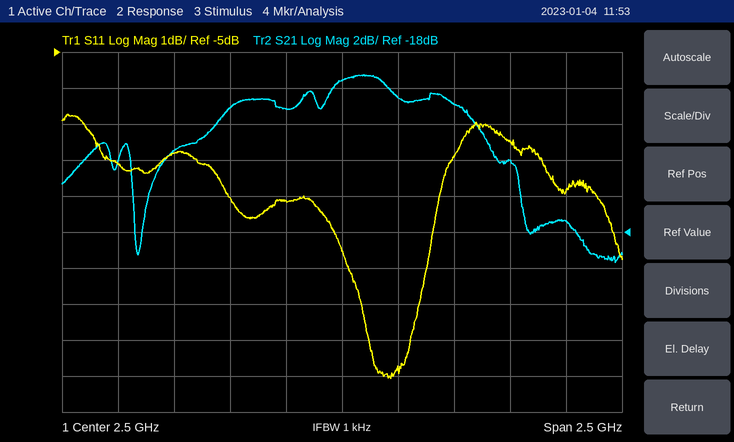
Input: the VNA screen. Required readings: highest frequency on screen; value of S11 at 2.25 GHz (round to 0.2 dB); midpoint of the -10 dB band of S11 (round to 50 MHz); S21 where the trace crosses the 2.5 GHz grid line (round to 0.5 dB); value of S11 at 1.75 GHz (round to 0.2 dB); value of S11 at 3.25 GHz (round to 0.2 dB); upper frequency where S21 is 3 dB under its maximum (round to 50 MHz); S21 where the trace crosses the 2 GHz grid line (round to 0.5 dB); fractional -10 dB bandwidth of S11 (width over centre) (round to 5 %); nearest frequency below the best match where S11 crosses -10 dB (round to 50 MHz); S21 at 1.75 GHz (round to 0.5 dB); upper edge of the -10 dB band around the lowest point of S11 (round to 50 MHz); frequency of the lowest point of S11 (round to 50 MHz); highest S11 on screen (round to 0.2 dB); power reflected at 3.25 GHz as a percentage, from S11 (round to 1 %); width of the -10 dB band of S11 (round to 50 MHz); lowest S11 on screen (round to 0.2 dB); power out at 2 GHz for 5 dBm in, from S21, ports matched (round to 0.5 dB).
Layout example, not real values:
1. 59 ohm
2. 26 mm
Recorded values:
1. 3.75 GHz
2. -9.2 dB
3. 2.70 GHz
4. -9.5 dB
5. -7.8 dB
6. -7.4 dB
7. 3.10 GHz
8. -11.0 dB
9. 15 %
10. 2.45 GHz
11. -13.5 dB
12. 2.90 GHz
13. 2.70 GHz
14. -6.8 dB
15. 18 %
16. 450 MHz
17. -14.0 dB
18. -6.0 dBm
